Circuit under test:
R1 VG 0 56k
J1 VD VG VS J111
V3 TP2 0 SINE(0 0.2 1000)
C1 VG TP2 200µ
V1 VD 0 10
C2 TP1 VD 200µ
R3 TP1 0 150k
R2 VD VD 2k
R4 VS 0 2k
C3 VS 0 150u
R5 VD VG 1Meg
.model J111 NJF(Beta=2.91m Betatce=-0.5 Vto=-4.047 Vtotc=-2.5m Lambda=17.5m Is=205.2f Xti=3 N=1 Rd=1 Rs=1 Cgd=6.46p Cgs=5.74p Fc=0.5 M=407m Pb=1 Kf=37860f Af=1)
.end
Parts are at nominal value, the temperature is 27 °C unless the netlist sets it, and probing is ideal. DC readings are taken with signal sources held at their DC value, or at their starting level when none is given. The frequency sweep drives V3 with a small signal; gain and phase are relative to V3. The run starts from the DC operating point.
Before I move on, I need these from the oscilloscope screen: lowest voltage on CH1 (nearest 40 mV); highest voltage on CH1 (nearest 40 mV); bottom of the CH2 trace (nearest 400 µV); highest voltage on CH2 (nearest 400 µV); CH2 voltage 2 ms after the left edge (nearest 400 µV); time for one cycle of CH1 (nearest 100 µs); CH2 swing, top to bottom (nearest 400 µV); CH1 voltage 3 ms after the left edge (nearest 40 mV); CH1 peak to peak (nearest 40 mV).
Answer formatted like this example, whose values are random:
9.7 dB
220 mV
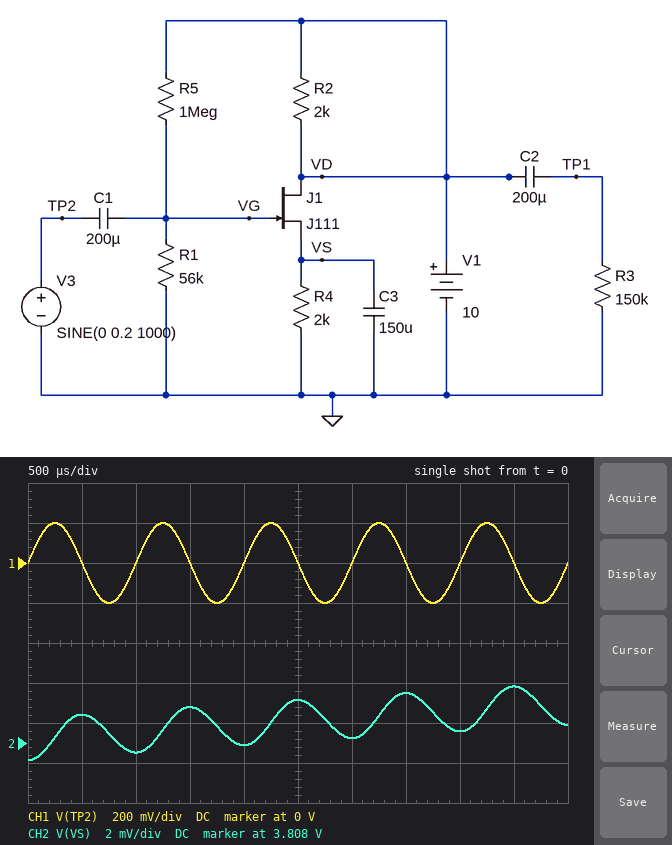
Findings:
-200 mV
200 mV
3.8072 V
3.8108 V
3.8080 V
1.0 ms
3.6 mV
0 V
400 mV
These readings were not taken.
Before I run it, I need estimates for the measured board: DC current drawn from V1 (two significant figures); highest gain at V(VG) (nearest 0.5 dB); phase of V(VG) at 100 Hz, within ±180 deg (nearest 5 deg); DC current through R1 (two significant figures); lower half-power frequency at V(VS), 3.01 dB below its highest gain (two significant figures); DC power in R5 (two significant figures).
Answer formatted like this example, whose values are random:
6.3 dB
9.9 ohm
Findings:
1.9 mA
0 dB
0 deg
9.5 µA
15 mHz
90 µW
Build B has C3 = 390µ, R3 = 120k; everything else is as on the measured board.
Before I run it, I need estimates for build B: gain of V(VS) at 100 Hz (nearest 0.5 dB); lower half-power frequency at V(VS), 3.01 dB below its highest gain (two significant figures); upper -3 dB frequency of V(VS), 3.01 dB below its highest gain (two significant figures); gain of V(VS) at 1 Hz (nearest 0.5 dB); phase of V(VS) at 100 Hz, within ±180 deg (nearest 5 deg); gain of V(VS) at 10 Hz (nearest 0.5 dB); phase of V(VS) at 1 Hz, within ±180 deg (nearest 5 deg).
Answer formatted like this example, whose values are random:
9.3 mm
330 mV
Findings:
-34.0 dB
15 mHz
2.3 Hz
-1.5 dB
-90 deg
-14.0 dB
-25 deg
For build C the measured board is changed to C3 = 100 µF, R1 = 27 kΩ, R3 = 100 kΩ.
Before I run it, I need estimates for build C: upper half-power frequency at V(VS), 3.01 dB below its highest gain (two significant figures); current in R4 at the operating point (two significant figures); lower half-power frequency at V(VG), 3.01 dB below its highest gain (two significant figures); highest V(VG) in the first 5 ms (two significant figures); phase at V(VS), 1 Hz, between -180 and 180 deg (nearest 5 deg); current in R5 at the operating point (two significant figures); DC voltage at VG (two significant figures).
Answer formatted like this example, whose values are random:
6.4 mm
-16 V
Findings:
8.5 Hz
1.8 mA
30 mHz
460 mV
-5 deg
9.7 µA
260 mV
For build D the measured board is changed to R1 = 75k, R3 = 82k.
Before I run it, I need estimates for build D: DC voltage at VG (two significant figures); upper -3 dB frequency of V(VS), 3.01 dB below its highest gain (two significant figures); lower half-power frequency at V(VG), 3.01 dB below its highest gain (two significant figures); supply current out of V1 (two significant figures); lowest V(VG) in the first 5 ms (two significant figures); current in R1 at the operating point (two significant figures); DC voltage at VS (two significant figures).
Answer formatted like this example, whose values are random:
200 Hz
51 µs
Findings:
700 mV
5.9 Hz
11 mHz
2.0 mA
500 mV
9.3 µA
4.0 V
